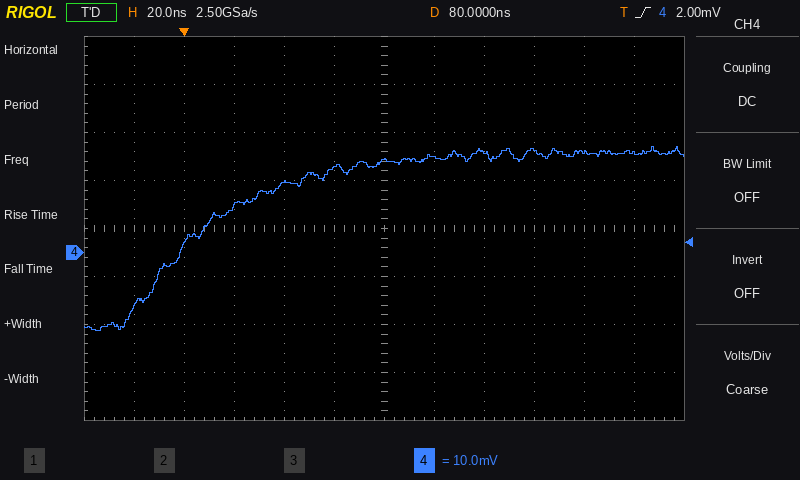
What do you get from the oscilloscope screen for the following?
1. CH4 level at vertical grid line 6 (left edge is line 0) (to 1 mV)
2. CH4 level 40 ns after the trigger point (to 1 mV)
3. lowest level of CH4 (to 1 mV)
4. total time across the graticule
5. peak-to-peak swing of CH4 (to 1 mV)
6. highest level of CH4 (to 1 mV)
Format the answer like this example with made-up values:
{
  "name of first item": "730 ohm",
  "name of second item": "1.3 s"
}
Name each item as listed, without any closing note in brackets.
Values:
{
  "CH4 level at vertical grid line 6 (left edge is line 0)": "19 mV",
  "CH4 level 40 ns after the trigger point": "15 mV",
  "lowest level of CH4": "-16 mV",
  "total time across the graticule": "240 ns",
  "peak-to-peak swing of CH4": "38 mV",
  "highest level of CH4": "22 mV"
}
